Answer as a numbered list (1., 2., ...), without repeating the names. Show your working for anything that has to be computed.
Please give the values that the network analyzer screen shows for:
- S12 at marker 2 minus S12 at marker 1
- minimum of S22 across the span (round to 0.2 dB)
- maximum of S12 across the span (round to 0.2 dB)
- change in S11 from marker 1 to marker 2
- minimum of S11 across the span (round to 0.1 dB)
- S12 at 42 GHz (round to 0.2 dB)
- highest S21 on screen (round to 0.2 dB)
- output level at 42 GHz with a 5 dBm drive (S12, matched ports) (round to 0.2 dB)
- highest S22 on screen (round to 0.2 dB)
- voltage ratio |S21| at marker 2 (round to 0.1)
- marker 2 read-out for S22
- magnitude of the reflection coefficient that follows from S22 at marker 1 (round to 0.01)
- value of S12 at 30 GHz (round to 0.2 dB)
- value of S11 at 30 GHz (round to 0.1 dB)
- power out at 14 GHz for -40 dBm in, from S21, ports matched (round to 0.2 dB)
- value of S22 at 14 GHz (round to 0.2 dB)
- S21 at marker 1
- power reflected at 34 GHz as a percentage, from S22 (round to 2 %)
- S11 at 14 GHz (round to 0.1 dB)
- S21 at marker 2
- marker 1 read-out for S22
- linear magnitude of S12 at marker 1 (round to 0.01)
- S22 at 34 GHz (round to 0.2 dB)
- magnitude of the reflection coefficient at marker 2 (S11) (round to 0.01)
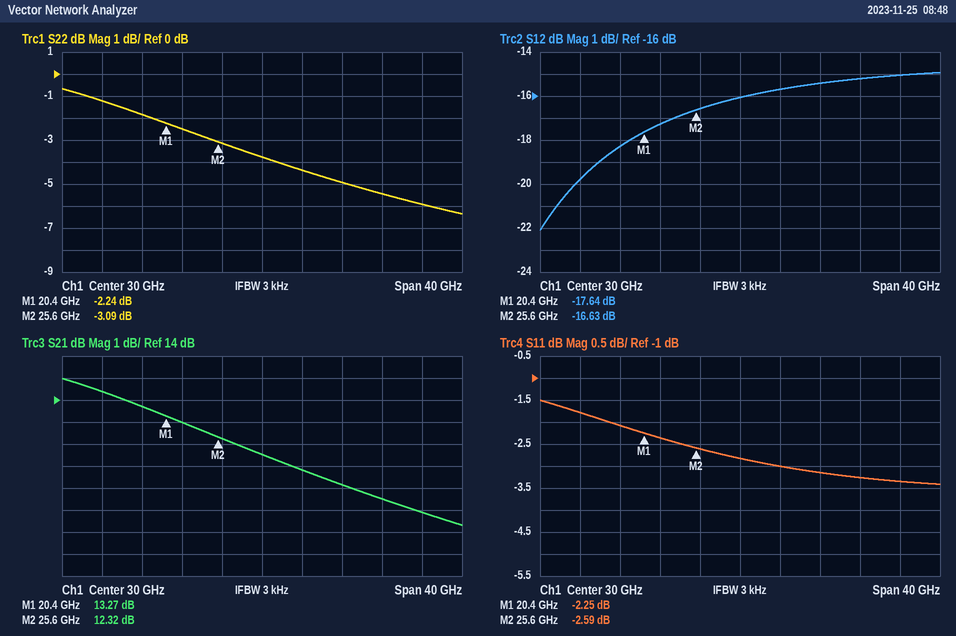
1. -16.63 − (-17.64) = 1.01 dB
2. -6.4 dB
3. -15.0 dB
4. -2.59 − (-2.25) = -0.34 dB
5. -3.4 dB
6. -15.2 dB
7. 15.0 dB
8. 5 dBm + (-15.2 dB) = -10.2 dBm
9. -0.6 dB
10. 10^(12.32/20) ≈ 4.1
11. -3.09 dB
12. 10^(-2.24/20) ≈ 0.77
13. -16.0 dB
14. -2.8 dB
15. -40 dBm + (14.4 dB) = -25.6 dBm
16. -1.2 dB
17. 13.27 dB
18. 10^(-4.4/10) ≈ 36 %
19. -1.8 dB
20. 12.32 dB
21. -2.24 dB
22. 10^(-17.64/20) ≈ 0.13
23. -4.4 dB
24. 10^(-2.59/20) ≈ 0.74
